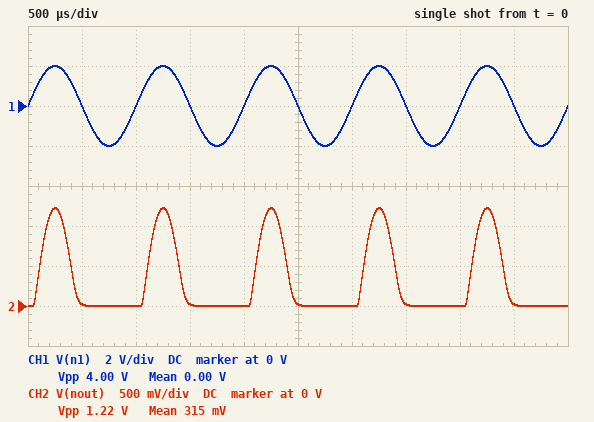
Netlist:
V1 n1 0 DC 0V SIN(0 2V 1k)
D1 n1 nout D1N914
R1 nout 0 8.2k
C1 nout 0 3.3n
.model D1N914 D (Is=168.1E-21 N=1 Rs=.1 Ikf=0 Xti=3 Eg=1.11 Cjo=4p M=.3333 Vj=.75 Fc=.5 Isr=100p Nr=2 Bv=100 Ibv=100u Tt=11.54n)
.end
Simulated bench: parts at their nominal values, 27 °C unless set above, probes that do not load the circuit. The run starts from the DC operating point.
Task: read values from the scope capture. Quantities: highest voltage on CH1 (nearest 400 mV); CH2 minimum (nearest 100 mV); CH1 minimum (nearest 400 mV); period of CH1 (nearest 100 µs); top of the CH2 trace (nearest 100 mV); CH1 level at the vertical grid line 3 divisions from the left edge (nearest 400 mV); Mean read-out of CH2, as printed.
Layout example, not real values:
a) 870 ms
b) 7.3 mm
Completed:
a) 2.0 V
b) 0 V
c) -2.0 V
d) 1.0 ms
e) 1.2 V
f) 0 V
g) 315 mV
